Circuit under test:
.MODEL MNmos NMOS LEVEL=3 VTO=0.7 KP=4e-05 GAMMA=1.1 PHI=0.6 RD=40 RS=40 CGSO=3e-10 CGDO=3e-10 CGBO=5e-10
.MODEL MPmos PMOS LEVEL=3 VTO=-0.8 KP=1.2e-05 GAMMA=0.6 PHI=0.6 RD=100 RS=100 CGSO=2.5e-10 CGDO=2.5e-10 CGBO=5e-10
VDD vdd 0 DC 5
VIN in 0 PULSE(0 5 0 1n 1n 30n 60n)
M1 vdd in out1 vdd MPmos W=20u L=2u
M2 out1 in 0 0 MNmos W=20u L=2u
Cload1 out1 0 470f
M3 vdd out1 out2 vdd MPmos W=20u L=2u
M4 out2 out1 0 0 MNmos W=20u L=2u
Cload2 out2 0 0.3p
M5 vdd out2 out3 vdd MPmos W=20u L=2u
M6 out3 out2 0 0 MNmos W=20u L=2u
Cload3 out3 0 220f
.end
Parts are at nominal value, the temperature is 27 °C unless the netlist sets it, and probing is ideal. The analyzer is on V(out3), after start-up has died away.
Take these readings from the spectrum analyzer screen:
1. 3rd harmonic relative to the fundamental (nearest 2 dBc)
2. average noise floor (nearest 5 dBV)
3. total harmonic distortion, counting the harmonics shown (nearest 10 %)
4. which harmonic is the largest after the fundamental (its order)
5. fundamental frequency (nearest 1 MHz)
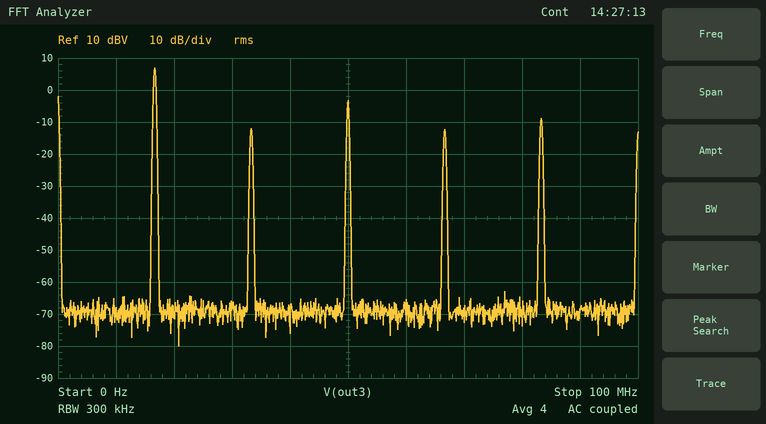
-10 dBc
-70 dBV
40 %
3
17 MHz
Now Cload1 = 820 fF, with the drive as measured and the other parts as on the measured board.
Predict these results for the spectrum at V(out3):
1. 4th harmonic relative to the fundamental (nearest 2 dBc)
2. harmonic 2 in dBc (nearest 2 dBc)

-18 dBc
-16 dBc
